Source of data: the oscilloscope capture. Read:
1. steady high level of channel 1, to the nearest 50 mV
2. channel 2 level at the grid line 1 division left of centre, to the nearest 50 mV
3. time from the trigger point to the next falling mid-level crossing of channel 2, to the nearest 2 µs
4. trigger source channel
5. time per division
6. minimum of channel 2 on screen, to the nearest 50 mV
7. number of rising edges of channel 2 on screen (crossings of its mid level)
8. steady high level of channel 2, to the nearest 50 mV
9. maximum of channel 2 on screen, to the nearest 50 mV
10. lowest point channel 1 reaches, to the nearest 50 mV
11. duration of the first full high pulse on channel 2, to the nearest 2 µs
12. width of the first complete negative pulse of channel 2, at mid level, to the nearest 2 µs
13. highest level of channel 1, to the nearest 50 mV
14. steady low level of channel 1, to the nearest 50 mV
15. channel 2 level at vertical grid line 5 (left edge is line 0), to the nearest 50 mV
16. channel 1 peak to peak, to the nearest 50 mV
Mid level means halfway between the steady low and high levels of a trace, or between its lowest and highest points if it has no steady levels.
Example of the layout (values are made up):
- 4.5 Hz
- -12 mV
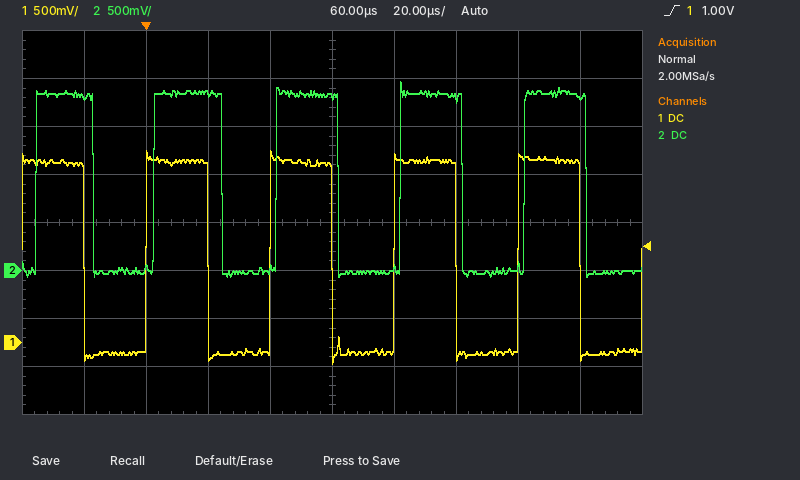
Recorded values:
- 1.90 V
- 0 mV
- 24 µs
- channel 1
- 20 µs
- -50 mV
- 5
- 1.85 V
- 1.95 V
- -200 mV
- 18 µs
- 20 µs
- 2.00 V
- -100 mV
- 1.80 V
- 2.20 V
